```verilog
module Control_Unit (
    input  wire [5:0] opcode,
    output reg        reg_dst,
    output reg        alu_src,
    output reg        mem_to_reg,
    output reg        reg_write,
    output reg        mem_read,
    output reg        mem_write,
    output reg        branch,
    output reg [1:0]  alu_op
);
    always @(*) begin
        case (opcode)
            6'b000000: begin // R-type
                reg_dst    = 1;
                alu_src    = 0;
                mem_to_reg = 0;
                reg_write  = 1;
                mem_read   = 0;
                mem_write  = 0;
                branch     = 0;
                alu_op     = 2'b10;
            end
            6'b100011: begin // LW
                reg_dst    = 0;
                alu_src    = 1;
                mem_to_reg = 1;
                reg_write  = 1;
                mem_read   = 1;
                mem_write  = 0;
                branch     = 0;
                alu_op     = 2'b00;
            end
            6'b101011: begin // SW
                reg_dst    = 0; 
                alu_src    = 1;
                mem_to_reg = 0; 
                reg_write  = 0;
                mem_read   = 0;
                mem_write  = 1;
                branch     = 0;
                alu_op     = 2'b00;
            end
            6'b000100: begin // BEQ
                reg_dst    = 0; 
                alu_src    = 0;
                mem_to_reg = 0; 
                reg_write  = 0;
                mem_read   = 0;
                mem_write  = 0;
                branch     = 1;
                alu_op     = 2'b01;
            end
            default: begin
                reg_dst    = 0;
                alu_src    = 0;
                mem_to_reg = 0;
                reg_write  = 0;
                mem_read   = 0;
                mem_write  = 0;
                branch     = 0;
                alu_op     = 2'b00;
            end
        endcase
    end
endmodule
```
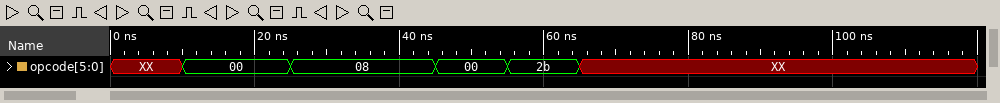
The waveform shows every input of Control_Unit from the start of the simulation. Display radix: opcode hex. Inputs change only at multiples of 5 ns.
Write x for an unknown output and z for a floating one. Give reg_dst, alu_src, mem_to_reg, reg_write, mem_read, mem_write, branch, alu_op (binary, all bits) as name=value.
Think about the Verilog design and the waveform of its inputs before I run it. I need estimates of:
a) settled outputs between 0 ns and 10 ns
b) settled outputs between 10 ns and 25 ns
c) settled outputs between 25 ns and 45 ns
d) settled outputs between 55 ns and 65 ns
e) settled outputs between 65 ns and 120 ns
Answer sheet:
reg_dst=x, alu_src=x, mem_to_reg=x, reg_write=x, mem_read=x, mem_write=x, branch=x, alu_op=x
reg_dst=1, alu_src=0, mem_to_reg=0, reg_write=1, mem_read=0, mem_write=0, branch=0, alu_op=10
reg_dst=0, alu_src=0, mem_to_reg=0, reg_write=0, mem_read=0, mem_write=0, branch=0, alu_op=00
reg_dst=0, alu_src=1, mem_to_reg=0, reg_write=0, mem_read=0, mem_write=1, branch=0, alu_op=00
reg_dst=0, alu_src=0, mem_to_reg=0, reg_write=0, mem_read=0, mem_write=0, branch=0, alu_op=00
